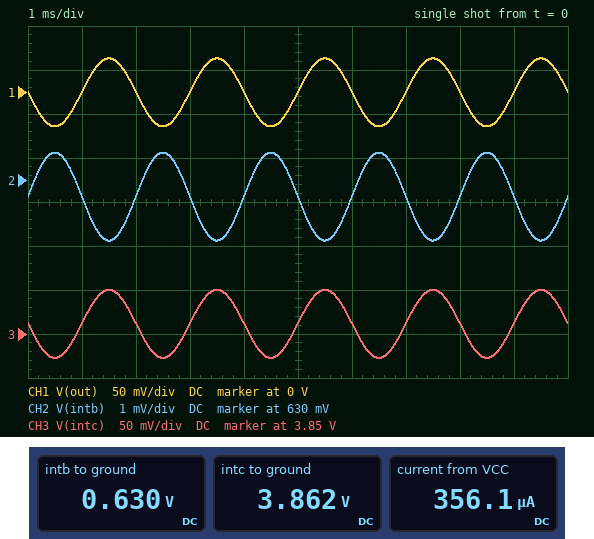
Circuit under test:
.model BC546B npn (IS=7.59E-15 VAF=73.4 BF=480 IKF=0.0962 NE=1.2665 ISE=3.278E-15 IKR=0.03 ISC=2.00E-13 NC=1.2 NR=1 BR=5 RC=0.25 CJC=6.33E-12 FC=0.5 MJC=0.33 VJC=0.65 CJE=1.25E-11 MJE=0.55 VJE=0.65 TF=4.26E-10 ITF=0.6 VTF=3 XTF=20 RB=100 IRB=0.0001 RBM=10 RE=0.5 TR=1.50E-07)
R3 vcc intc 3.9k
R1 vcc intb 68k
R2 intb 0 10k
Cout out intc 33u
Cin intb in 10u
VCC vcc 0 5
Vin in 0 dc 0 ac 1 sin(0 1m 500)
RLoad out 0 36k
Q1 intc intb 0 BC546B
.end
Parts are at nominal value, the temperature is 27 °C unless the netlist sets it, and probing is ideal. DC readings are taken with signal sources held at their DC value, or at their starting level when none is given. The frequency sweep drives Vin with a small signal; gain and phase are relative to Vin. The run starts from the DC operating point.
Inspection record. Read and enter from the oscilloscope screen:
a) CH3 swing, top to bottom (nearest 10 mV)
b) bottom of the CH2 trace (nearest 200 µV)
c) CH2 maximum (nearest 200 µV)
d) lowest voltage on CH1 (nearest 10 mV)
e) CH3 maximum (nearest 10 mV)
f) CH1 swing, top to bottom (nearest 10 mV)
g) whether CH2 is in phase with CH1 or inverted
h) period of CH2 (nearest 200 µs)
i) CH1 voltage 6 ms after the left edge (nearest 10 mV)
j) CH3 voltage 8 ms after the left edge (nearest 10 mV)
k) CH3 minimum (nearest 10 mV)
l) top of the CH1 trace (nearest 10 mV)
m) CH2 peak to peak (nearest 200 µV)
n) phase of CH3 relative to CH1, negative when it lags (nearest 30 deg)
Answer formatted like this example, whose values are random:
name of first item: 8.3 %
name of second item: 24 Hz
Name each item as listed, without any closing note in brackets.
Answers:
CH3 swing, top to bottom: 80 mV
bottom of the CH2 trace: 628.6 mV
CH2 maximum: 630.6 mV
lowest voltage on CH1: -40 mV
CH3 maximum: 3.90 V
CH1 swing, top to bottom: 80 mV
whether CH2 is in phase with CH1 or inverted: inverted
period of CH2: 2.0 ms
CH1 voltage 6 ms after the left edge: 0 V
CH3 voltage 8 ms after the left edge: 3.86 V
CH3 minimum: 3.82 V
top of the CH1 trace: 40 mV
CH2 peak to peak: 2.0 mV
phase of CH3 relative to CH1, negative when it lags: 0 deg
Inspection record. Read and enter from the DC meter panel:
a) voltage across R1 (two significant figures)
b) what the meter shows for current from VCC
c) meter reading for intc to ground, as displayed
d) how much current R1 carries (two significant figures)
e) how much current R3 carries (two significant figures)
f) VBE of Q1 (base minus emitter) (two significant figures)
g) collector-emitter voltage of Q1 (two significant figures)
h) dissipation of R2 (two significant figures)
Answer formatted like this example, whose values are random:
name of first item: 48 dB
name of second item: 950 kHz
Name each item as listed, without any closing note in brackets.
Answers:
voltage across R1: 4.4 V
what the meter shows for current from VCC: 356.1 µA
meter reading for intc to ground, as displayed: 3.862 V
how much current R1 carries: 64 µA
how much current R3 carries: 290 µA
VBE of Q1 (base minus emitter): 630 mV
collector-emitter voltage of Q1: 3.9 V
dissipation of R2: 40 µW
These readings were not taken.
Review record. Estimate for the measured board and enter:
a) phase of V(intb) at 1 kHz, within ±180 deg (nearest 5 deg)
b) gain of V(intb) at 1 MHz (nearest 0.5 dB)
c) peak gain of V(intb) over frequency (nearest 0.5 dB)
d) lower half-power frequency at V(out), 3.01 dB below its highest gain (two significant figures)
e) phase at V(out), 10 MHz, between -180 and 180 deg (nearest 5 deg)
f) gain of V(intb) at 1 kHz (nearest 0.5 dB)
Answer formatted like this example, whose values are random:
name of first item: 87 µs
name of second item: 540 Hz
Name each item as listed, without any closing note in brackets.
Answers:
phase of V(intb) at 1 kHz, within ±180 deg: 0 deg
gain of V(intb) at 1 MHz: 0 dB
peak gain of V(intb) over frequency: 0 dB
lower half-power frequency at V(out), 3.01 dB below its highest gain: 2.5 Hz
phase at V(out), 10 MHz, between -180 and 180 deg: 115 deg
gain of V(intb) at 1 kHz: 0 dB
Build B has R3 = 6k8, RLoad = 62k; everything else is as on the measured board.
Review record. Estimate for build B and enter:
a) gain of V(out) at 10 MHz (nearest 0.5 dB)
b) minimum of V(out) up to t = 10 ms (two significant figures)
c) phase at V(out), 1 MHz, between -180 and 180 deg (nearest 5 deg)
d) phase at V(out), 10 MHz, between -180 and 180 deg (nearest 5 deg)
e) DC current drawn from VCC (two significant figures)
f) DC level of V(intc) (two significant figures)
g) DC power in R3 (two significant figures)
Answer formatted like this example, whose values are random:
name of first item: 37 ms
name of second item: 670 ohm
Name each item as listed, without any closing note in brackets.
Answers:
gain of V(out) at 10 MHz: 26.0 dB
minimum of V(out) up to t = 10 ms: -67 mV
phase at V(out), 1 MHz, between -180 and 180 deg: 160 deg
phase at V(out), 10 MHz, between -180 and 180 deg: 100 deg
DC current drawn from VCC: 350 µA
DC level of V(intc): 3.0 V
DC power in R3: 570 µW
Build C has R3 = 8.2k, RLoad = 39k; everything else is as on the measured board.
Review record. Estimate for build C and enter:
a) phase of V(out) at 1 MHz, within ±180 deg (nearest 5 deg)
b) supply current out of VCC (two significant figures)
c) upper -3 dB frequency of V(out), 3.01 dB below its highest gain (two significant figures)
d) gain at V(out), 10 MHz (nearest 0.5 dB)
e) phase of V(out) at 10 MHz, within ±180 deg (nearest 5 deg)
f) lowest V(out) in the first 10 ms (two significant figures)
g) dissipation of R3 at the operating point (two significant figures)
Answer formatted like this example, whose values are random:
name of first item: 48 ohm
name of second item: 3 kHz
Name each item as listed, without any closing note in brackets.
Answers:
phase of V(out) at 1 MHz, within ±180 deg: 160 deg
supply current out of VCC: 350 µA
upper -3 dB frequency of V(out), 3.01 dB below its highest gain: 2.8 MHz
gain at V(out), 10 MHz: 26.0 dB
phase of V(out) at 10 MHz, within ±180 deg: 100 deg
lowest V(out) in the first 10 ms: -73 mV
dissipation of R3 at the operating point: 680 µW
